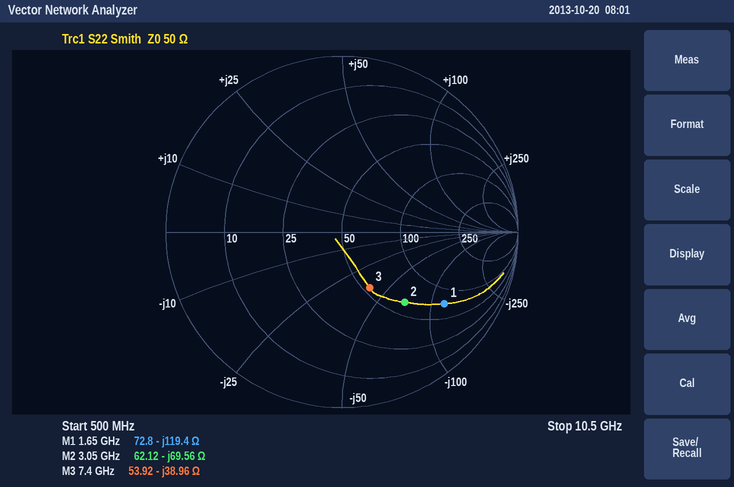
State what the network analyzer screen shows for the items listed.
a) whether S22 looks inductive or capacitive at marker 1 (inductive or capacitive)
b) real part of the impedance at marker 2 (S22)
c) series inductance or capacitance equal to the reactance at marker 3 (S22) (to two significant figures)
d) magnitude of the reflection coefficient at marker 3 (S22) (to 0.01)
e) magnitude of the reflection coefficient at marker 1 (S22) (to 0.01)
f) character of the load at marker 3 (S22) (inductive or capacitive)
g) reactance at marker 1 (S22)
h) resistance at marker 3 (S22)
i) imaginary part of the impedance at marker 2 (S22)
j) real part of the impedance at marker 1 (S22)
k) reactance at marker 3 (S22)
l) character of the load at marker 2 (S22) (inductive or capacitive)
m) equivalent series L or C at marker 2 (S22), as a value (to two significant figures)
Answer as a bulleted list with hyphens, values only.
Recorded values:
- capacitive
- 62.12 Ω
- 550 fF
- 0.35
- 0.71
- capacitive
- -119.4 Ω
- 53.92 Ω
- -69.56 Ω
- 72.8 Ω
- -38.96 Ω
- capacitive
- 750 fF
